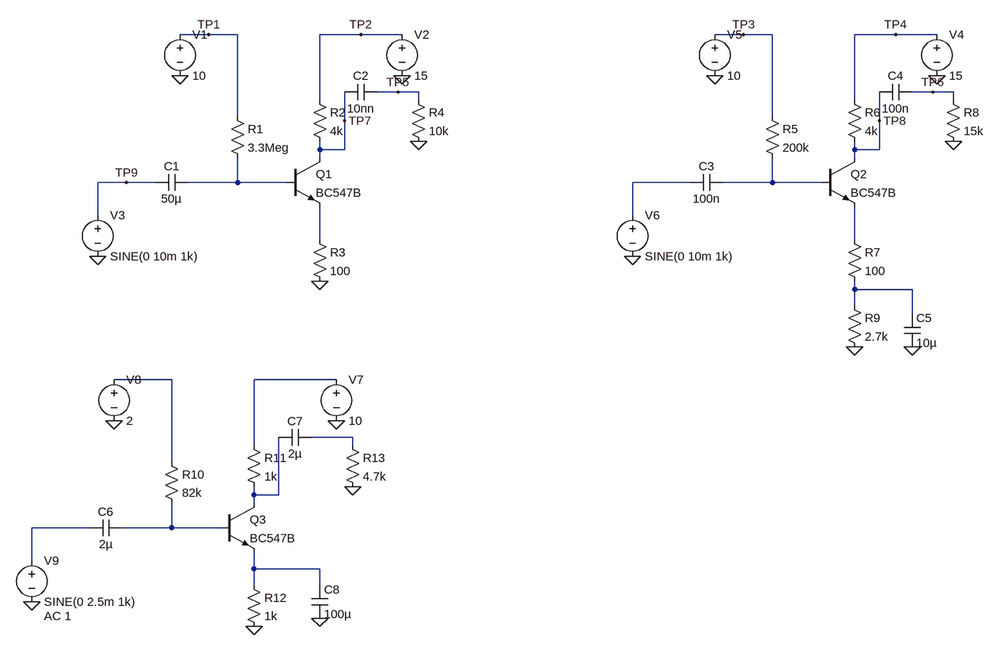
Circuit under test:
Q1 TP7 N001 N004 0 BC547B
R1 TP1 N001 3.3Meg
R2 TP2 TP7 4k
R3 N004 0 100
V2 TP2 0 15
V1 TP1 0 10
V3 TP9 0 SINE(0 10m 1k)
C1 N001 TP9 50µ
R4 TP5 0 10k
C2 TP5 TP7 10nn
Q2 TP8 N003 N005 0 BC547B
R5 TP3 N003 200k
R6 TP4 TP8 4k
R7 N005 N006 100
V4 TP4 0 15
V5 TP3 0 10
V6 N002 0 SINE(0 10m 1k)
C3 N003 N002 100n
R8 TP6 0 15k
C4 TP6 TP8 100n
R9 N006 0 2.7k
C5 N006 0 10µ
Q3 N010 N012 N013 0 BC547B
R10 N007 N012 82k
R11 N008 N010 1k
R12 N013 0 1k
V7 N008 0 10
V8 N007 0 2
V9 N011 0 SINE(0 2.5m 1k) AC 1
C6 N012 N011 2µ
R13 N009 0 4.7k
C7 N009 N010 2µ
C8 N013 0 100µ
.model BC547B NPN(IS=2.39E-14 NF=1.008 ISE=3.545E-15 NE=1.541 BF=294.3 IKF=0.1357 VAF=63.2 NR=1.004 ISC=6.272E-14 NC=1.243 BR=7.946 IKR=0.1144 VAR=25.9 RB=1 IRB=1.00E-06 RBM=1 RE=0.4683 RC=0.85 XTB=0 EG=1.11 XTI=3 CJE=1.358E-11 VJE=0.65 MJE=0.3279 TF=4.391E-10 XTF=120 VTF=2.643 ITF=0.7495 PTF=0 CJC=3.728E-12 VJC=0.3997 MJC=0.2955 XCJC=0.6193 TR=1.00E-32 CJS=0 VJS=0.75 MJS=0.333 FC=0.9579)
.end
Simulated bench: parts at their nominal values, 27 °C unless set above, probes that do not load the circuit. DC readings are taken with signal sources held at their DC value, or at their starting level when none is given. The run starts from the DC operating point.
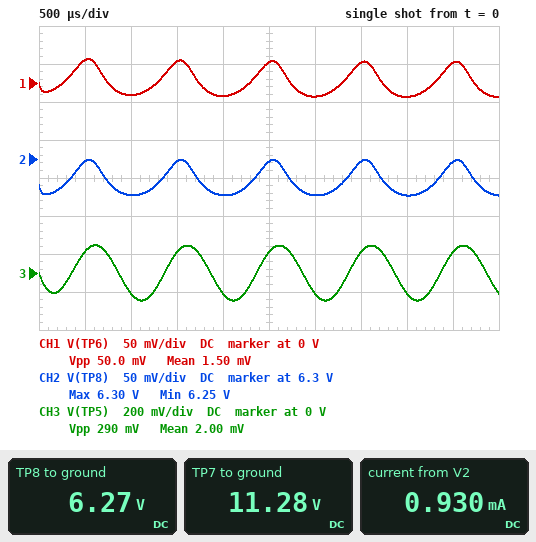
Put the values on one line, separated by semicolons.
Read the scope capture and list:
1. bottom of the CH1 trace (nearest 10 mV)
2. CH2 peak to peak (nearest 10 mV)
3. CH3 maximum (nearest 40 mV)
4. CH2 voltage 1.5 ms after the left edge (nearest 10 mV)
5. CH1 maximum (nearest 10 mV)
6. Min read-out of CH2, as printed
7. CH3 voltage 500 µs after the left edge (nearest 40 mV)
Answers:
-20 mV; 50 mV; 160 mV; 6.30 V; 30 mV; 6.25 V; 120 mV
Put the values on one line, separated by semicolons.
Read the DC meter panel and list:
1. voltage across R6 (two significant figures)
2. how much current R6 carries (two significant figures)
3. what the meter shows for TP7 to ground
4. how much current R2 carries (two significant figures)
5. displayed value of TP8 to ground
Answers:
8.7 V; 2.2 mA; 11.28 V; 930 µA; 6.27 V
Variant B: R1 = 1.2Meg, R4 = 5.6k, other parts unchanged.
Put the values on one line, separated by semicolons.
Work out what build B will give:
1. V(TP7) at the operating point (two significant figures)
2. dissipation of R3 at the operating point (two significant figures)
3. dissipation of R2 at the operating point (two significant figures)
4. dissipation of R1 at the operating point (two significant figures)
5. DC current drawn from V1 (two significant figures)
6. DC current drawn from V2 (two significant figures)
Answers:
5.8 V; 530 µW; 21 mW; 69 µW; 7.6 µA; 2.3 mA
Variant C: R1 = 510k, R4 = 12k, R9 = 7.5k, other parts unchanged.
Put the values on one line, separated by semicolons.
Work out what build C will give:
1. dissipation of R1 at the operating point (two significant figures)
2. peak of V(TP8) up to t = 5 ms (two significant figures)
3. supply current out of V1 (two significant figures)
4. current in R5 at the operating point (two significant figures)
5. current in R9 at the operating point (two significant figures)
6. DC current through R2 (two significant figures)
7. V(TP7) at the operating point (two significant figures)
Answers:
160 µW; 11 V; 18 µA; 3.9 µA; 1.1 mA; 3.6 mA; 500 mV
